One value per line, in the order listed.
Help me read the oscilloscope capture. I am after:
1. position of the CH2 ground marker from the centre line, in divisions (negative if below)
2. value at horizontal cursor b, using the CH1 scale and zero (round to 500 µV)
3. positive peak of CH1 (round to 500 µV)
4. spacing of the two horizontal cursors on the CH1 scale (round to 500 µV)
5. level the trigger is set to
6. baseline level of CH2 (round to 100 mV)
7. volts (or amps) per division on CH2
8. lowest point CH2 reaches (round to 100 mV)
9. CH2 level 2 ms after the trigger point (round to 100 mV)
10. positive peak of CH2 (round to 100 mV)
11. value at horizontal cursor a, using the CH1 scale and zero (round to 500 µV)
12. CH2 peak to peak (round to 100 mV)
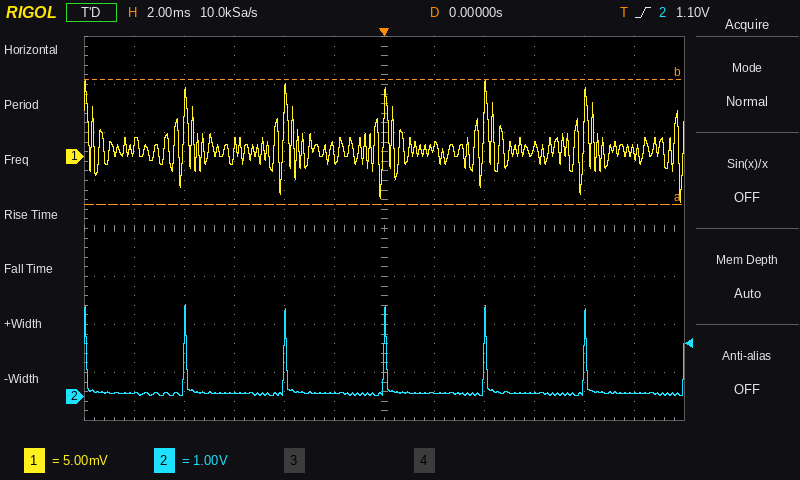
-3.5 div
8.0 mV
8.0 mV
13.0 mV
1.10 V
100 mV
1 V
0.0 V
100 mV
1.9 V
-5.0 mV
1.9 V
